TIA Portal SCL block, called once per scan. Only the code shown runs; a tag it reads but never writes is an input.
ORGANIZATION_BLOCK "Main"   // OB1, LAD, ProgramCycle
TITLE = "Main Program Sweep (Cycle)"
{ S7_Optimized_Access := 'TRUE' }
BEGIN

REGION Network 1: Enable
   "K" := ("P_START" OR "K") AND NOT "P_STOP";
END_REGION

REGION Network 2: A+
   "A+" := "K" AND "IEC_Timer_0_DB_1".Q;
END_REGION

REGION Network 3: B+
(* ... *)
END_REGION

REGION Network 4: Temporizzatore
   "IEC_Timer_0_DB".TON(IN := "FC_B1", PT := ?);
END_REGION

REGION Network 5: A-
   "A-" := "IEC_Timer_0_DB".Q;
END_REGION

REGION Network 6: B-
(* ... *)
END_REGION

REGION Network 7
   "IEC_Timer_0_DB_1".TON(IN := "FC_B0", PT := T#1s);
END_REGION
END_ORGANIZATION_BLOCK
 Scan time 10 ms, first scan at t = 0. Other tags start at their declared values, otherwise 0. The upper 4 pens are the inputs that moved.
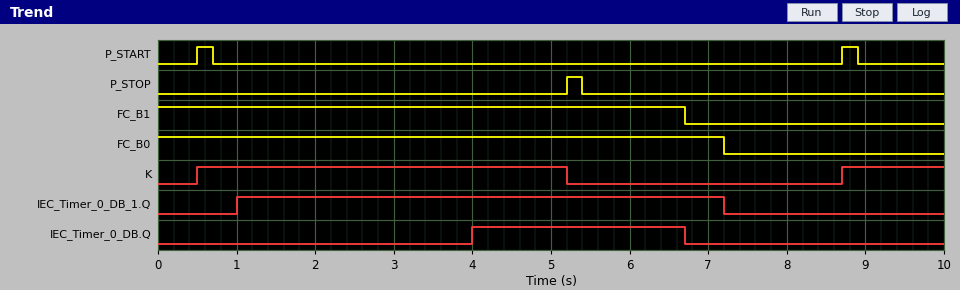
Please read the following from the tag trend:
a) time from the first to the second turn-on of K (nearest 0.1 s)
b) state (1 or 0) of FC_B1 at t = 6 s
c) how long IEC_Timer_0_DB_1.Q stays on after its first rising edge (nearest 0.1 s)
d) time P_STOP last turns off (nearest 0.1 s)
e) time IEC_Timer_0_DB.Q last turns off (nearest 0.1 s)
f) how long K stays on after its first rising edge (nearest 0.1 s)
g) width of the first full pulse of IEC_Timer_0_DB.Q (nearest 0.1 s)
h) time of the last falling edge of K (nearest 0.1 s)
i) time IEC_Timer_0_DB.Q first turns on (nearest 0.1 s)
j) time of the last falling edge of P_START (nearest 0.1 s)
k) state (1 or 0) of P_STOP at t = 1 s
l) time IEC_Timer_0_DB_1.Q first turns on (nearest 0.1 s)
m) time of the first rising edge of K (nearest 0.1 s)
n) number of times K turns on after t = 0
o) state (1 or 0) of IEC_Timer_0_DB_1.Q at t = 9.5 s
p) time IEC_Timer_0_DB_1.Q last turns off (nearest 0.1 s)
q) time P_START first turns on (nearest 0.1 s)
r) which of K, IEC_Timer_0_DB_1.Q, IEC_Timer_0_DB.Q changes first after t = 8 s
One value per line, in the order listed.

8.2 s
1
6.2 s
5.4 s
6.7 s
4.7 s
2.7 s
5.2 s
4.0 s
8.9 s
0
1.0 s
0.5 s
2
0
7.2 s
0.5 s
K
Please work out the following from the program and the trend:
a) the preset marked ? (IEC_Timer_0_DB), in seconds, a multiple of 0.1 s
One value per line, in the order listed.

4.0 s
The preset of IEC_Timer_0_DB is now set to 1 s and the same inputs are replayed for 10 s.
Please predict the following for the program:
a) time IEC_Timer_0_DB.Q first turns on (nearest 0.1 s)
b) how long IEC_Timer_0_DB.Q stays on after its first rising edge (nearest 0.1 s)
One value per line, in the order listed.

1.0 s
5.7 s
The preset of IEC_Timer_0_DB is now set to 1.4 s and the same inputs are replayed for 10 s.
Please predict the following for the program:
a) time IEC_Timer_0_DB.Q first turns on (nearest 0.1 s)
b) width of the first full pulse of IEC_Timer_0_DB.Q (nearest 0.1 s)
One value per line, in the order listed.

1.4 s
5.3 s
